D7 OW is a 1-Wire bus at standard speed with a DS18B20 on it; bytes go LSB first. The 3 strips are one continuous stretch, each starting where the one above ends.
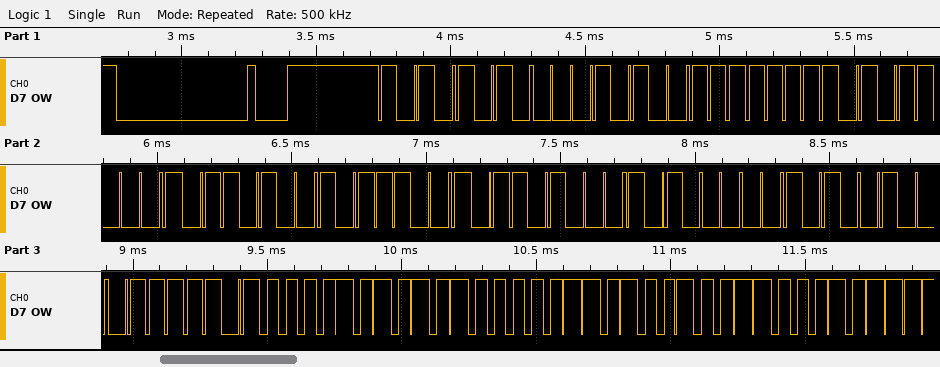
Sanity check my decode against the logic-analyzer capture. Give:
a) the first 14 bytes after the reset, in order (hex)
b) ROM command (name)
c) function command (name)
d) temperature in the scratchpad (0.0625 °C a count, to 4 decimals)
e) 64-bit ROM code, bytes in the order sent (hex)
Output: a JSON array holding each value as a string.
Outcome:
["55 28 FF 1A 2D 9D 16 05 25 BE 50 05 4B 46", "Match ROM", "Read Scratchpad", "85.0000 °C", "28 FF 1A 2D 9D 16 05 25"]
